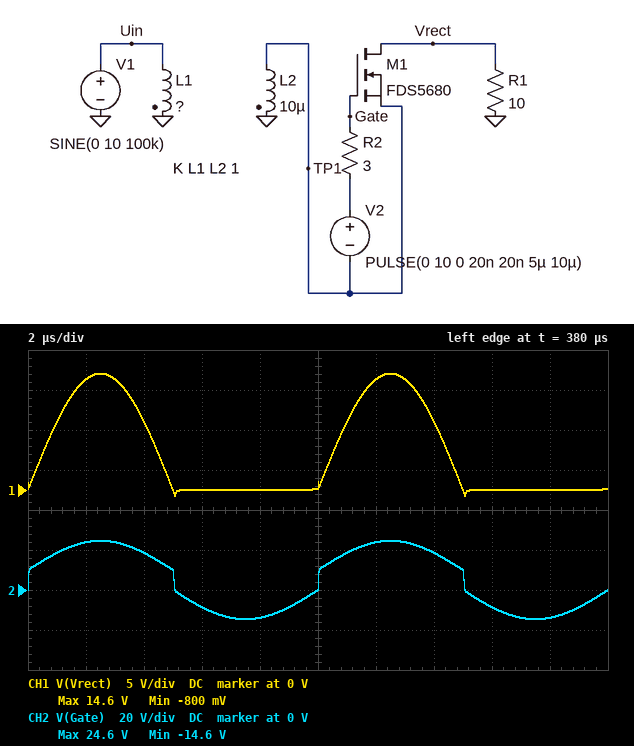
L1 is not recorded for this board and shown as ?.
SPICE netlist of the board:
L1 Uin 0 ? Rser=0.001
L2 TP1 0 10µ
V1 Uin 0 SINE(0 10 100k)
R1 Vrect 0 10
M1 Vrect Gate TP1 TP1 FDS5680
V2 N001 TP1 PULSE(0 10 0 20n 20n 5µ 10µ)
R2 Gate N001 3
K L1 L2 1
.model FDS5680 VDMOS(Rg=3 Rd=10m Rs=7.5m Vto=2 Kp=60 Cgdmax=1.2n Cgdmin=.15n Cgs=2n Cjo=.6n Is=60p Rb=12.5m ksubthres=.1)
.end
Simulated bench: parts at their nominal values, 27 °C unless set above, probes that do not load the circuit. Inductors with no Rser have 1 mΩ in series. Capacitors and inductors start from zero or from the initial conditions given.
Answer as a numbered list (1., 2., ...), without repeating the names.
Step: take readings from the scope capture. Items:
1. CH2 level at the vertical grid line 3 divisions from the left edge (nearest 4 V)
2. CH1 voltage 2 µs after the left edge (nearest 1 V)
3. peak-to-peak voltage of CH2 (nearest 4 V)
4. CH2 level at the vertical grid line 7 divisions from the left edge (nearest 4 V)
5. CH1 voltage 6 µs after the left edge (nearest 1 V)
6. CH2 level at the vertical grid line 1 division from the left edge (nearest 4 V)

1. -8 V
2. 14 V
3. 40 V
4. 20 V
5. 0 V
6. 24 V
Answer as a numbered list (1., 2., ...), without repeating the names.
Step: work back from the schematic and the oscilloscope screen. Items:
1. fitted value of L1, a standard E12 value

1. 4.7 µH
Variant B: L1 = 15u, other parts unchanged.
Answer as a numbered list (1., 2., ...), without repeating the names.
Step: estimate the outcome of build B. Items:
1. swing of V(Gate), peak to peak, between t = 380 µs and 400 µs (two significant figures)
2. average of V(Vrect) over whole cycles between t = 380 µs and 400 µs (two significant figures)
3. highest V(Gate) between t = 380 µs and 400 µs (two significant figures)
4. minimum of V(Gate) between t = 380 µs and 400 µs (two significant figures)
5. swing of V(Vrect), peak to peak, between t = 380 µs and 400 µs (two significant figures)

1. 26 V
2. 2.6 V
3. 18 V
4. -8.2 V
5. 8.8 V
